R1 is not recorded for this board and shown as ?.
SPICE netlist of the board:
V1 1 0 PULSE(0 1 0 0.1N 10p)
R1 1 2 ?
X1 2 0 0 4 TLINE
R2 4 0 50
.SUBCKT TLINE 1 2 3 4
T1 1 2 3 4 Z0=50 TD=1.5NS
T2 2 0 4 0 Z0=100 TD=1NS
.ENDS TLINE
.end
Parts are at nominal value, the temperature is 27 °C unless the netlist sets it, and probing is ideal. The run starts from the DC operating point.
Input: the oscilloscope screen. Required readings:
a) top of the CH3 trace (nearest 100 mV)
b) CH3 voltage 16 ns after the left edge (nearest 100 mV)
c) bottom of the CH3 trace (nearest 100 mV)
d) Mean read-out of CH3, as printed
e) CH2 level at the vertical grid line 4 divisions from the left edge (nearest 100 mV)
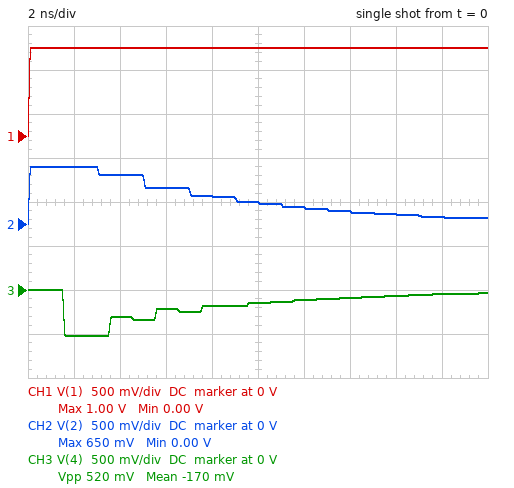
0 V
-100 mV
-500 mV
-170 mV
300 mV
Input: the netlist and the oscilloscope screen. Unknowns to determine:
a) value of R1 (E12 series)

27 Ω
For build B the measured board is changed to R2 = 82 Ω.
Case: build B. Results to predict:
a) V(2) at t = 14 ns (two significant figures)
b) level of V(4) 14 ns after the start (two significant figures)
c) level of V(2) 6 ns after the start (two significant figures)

140 mV
-82 mV
420 mV
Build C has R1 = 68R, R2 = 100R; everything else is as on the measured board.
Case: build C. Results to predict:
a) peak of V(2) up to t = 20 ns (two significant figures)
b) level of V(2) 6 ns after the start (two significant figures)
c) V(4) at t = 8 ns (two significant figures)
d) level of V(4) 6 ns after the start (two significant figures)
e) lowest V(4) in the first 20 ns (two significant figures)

420 mV
180 mV
-21 mV
-110 mV
-420 mV
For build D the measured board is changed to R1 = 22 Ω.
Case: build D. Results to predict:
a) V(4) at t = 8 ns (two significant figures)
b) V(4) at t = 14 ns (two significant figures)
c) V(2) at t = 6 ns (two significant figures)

-220 mV
-120 mV
470 mV
